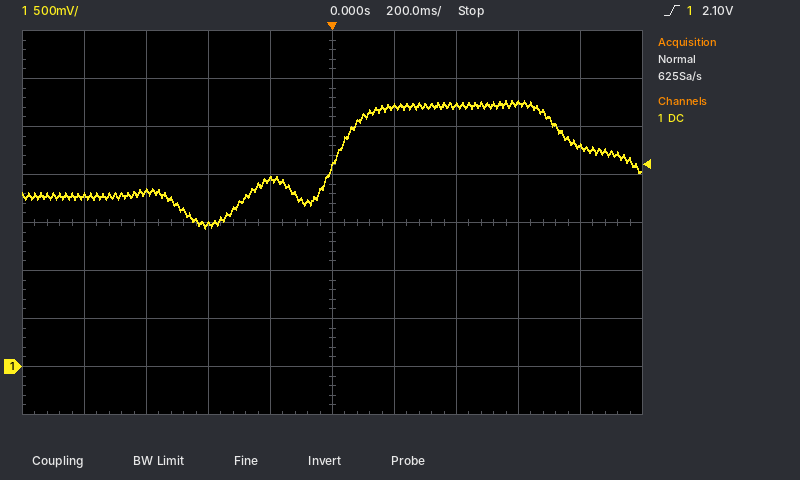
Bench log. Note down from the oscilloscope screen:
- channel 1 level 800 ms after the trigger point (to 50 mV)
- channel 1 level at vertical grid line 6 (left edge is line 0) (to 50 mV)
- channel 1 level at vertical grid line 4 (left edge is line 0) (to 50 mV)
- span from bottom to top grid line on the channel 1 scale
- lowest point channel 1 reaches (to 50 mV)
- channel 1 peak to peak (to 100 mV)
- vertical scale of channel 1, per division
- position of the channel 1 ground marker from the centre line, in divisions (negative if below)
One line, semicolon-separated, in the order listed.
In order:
2.30 V; 2.70 V; 1.95 V; 4 V; 1.45 V; 1.30 V; 500 mV; -3.0 div
